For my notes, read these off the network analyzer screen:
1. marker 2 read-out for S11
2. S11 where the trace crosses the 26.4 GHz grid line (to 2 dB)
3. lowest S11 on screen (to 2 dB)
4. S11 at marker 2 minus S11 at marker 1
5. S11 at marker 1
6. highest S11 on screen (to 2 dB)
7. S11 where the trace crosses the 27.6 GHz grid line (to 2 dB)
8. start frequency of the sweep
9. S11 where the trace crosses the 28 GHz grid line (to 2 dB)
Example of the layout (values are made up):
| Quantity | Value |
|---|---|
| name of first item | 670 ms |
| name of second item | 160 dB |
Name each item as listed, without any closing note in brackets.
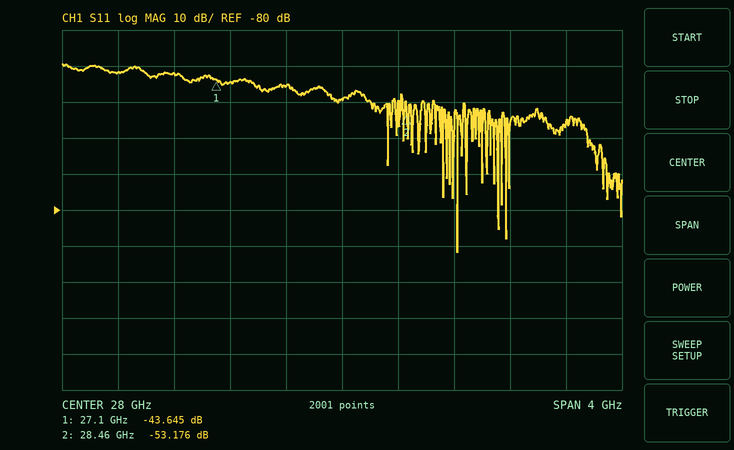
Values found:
| Quantity | Value |
|---|---|
| marker 2 read-out for S11 | -53.176 dB |
| S11 where the trace crosses the 26.4 GHz grid line | -42 dB |
| lowest S11 on screen | -92 dB |
| S11 at marker 2 minus S11 at marker 1 | -9.531 dB |
| S11 at marker 1 | -43.645 dB |
| highest S11 on screen | -40 dB |
| S11 where the trace crosses the 27.6 GHz grid line | -46 dB |
| start frequency of the sweep | 26 GHz |
| S11 where the trace crosses the 28 GHz grid line | -50 dB |
